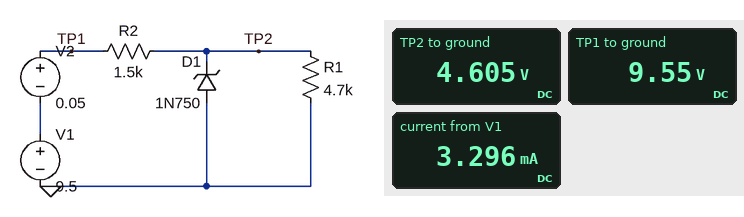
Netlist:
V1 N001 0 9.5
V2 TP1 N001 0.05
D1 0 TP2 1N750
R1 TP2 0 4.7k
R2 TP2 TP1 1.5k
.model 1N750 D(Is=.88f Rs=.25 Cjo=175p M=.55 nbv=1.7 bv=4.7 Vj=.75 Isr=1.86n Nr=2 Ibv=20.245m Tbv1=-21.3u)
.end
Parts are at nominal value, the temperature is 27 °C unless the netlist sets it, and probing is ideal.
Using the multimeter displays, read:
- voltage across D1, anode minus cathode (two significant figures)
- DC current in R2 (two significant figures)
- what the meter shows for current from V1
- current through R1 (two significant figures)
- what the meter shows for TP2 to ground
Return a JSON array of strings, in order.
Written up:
["-4.6 V", "3.3 mA", "3.296 mA", "980 µA", "4.605 V"]
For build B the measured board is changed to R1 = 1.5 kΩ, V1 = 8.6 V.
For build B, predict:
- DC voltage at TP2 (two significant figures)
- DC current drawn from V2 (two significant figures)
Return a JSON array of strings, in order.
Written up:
["4.3 V", "2.9 mA"]
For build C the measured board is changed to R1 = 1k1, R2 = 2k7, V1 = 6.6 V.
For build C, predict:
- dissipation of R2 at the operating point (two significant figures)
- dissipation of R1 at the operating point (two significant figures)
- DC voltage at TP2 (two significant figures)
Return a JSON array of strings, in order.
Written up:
["8.3 mW", "3.4 mW", "1.9 V"]
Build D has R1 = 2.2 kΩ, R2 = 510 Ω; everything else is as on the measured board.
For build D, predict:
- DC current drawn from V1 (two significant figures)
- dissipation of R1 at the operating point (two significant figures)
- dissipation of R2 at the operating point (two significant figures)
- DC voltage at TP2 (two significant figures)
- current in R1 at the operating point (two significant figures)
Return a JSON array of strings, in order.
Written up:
["9.6 mA", "9.9 mW", "47 mW", "4.7 V", "2.1 mA"]
